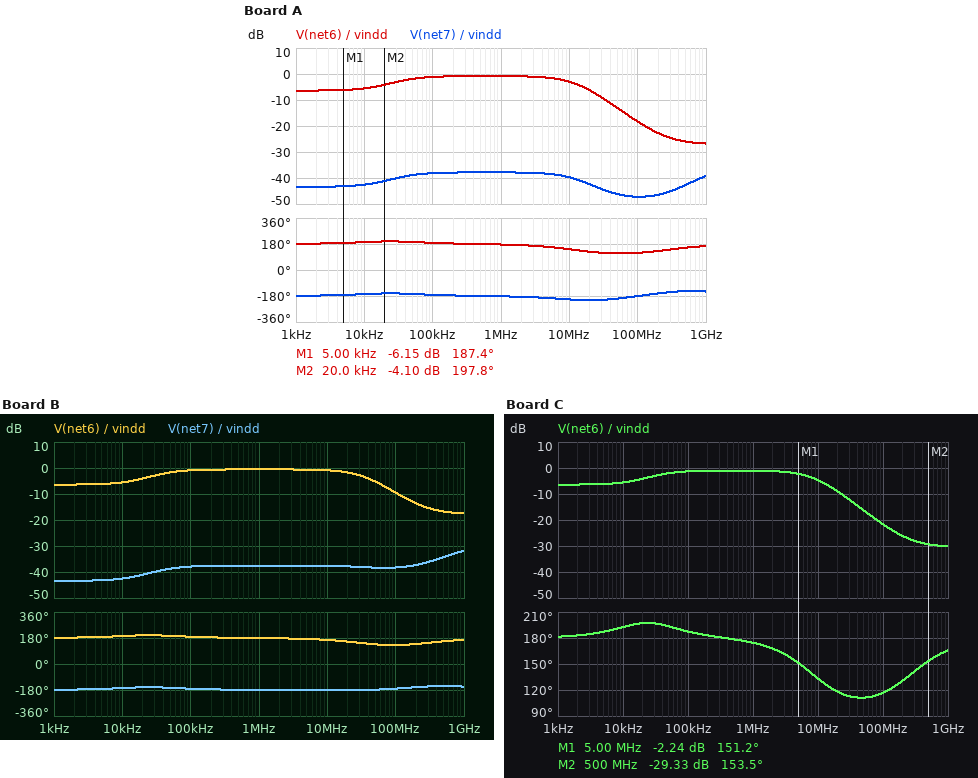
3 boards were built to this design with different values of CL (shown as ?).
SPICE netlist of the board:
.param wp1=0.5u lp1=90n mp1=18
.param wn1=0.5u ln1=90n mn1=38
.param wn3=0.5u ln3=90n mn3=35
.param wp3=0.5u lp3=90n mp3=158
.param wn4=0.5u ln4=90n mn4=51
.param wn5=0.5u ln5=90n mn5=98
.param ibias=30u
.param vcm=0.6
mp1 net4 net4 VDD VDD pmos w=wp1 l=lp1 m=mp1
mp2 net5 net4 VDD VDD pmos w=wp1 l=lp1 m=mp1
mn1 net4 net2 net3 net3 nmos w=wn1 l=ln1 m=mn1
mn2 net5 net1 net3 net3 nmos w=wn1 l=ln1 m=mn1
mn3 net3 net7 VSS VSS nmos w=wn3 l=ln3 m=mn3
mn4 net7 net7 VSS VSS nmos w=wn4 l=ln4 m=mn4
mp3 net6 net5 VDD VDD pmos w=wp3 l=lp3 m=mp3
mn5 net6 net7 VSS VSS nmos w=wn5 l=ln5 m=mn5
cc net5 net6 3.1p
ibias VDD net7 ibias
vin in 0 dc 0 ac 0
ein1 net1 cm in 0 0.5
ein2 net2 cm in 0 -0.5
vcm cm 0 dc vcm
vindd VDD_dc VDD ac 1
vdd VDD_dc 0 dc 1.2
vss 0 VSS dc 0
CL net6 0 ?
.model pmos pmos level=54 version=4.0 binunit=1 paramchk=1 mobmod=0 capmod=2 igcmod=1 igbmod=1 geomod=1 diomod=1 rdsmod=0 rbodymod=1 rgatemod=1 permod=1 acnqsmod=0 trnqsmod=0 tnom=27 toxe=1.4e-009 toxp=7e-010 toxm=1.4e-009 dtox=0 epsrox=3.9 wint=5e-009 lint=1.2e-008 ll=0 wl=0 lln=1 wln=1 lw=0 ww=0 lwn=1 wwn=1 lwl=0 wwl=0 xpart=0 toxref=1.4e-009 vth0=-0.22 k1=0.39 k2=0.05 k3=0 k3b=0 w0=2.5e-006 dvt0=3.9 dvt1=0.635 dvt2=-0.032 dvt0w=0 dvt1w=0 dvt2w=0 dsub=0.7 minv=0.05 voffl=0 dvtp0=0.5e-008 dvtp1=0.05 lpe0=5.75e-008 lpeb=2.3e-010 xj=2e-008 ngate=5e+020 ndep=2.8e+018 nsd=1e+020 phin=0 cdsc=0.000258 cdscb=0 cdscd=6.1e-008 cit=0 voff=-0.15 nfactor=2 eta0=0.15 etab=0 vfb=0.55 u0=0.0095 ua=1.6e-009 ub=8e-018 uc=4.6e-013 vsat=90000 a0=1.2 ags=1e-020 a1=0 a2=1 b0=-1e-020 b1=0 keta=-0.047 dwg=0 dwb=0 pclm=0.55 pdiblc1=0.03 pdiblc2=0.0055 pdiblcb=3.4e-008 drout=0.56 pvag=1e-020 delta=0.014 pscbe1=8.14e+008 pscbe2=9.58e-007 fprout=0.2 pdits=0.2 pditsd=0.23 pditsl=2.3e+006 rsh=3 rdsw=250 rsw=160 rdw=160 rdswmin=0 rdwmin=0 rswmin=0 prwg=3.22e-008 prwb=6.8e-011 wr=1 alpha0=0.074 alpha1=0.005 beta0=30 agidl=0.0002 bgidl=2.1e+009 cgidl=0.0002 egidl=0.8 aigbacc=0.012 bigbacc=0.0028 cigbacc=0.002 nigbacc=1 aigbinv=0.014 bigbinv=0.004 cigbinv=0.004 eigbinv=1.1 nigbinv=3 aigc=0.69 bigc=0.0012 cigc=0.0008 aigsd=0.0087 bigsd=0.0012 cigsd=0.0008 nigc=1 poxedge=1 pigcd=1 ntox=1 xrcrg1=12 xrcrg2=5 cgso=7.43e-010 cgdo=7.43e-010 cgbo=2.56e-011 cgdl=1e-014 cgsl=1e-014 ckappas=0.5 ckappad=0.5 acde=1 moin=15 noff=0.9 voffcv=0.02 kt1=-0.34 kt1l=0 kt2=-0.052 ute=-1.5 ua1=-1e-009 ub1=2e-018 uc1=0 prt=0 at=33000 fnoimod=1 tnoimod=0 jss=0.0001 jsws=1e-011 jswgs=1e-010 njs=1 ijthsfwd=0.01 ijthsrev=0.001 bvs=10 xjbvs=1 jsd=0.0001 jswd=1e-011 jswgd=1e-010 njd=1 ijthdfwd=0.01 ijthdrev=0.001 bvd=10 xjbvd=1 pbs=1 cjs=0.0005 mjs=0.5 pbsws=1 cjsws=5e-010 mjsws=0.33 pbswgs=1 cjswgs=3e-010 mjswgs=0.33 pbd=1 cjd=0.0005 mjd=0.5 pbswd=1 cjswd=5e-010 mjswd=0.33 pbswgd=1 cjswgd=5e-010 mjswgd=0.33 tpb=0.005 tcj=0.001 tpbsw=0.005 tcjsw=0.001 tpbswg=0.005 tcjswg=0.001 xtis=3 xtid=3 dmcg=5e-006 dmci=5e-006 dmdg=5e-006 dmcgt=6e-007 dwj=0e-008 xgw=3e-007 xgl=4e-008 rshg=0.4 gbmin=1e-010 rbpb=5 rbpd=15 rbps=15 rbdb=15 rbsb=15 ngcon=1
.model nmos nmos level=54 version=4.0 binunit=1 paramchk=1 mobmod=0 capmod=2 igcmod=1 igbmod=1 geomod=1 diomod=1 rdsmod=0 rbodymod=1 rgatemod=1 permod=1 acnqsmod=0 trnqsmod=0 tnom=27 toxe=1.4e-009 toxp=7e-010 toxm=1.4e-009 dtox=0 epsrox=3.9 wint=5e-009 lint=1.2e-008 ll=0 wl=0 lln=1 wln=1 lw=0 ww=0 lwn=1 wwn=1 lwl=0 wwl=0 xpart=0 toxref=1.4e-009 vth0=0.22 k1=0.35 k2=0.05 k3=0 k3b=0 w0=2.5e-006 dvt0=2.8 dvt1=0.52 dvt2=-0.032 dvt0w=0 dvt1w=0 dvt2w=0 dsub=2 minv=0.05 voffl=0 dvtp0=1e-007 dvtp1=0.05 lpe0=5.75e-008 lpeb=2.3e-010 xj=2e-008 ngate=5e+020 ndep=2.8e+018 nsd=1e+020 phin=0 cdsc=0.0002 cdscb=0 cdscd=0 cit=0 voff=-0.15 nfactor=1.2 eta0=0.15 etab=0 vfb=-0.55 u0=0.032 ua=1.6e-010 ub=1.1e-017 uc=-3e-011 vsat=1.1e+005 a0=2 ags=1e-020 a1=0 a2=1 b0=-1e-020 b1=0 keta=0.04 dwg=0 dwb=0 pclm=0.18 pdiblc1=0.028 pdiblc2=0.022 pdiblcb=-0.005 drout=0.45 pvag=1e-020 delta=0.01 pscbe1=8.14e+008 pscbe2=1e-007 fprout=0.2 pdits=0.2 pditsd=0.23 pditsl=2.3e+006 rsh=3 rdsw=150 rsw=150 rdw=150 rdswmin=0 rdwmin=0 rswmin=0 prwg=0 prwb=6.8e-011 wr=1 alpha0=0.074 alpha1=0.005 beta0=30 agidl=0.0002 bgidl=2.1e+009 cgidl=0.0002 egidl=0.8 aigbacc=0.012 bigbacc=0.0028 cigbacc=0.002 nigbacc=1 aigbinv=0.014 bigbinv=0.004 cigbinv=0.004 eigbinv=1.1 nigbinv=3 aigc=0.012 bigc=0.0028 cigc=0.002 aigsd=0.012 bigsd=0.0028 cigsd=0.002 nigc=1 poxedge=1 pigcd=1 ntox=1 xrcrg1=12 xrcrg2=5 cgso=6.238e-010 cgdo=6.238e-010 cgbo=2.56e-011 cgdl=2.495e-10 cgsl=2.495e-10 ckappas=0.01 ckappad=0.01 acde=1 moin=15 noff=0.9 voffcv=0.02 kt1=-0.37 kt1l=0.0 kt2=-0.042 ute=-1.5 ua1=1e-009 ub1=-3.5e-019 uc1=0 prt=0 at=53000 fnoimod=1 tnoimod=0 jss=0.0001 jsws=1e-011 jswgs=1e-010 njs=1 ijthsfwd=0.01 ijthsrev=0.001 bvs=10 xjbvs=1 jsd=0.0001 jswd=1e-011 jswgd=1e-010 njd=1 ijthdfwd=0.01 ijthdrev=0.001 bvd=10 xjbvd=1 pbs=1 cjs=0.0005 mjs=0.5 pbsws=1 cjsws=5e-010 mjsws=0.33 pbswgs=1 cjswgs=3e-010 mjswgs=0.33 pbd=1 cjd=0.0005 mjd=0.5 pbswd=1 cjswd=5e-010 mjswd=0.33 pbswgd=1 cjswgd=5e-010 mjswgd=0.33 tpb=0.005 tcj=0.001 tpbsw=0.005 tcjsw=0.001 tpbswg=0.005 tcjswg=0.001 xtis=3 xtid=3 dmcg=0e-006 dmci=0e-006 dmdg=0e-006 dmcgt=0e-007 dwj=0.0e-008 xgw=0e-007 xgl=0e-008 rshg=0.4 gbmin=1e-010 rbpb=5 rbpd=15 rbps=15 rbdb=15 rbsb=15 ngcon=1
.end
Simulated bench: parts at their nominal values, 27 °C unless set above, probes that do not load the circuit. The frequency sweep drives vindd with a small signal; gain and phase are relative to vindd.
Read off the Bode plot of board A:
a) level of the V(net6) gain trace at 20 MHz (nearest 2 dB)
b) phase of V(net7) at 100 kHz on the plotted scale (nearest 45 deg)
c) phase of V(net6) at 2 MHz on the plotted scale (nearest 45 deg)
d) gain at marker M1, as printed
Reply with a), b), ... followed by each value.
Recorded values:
a) -6 dB
b) -180 deg
c) 180 deg
d) -6.15 dB
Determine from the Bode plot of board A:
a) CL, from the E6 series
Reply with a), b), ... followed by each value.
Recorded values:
a) 22 pF
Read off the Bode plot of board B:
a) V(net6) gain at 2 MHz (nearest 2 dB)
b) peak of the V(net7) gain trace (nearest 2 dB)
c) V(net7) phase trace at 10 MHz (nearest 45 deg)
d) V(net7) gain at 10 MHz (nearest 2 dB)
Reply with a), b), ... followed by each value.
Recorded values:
a) 0 dB
b) -32 dB
c) -180 deg
d) -38 dB
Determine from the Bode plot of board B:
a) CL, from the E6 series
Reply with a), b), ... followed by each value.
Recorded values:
a) 6.8 pF
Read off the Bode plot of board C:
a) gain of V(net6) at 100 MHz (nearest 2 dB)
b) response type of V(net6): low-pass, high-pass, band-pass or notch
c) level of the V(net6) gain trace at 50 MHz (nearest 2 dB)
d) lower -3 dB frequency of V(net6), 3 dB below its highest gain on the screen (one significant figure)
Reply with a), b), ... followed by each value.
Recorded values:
a) -22 dB
b) low-pass
c) -16 dB
d) 20 kHz
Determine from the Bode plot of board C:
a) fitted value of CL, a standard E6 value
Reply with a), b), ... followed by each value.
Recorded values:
a) 33 pF
